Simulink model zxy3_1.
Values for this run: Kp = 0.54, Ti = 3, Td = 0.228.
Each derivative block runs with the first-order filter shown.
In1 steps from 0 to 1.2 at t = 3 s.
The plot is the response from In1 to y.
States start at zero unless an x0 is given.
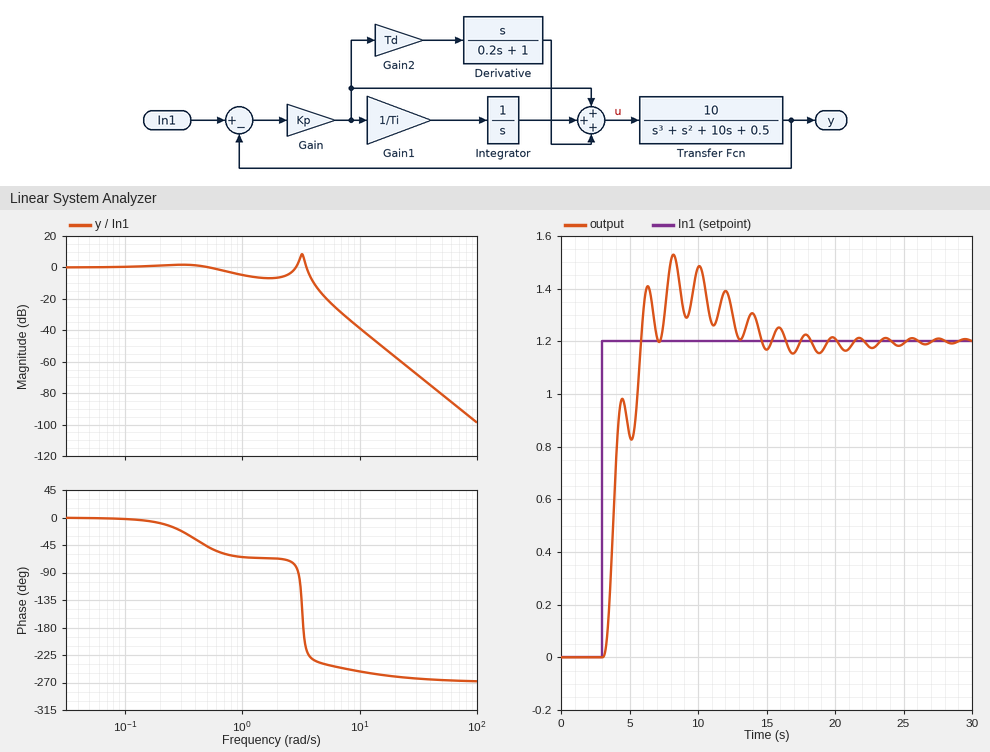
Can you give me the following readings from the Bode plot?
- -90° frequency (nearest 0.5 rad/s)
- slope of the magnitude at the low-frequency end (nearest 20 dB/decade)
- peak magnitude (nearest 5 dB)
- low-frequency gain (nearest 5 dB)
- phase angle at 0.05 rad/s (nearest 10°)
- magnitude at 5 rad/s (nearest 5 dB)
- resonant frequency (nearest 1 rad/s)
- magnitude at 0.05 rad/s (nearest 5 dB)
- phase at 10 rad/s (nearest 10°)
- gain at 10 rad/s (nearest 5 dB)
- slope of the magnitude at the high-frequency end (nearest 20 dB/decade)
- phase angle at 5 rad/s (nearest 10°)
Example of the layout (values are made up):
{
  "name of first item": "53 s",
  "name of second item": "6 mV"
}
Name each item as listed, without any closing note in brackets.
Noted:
{
  "-90° frequency": "3.0 rad/s",
  "slope of the magnitude at the low-frequency end": "0 dB/decade",
  "peak magnitude": "10 dB",
  "low-frequency gain": "0 dB",
  "phase angle at 0.05 rad/s": "0°",
  "magnitude at 5 rad/s": "-20 dB",
  "resonant frequency": "3 rad/s",
  "magnitude at 0.05 rad/s": "0 dB",
  "phase at 10 rad/s": "-250°",
  "gain at 10 rad/s": "-40 dB",
  "slope of the magnitude at the high-frequency end": "-60 dB/decade",
  "phase angle at 5 rad/s": "-240°"
}
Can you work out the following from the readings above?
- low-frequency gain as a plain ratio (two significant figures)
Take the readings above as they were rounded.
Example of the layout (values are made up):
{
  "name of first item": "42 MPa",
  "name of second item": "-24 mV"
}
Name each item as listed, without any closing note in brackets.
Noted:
{
  "low-frequency gain as a plain ratio": "1.0"
}
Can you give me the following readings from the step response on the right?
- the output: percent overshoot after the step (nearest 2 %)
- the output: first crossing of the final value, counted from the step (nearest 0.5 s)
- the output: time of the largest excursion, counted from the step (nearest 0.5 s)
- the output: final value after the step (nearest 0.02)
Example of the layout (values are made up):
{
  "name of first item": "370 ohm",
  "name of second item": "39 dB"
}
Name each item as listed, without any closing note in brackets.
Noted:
{
  "the output: percent overshoot after the step": "28 %",
  "the output: first crossing of the final value, counted from the step": "3.0 s",
  "the output: time of the largest excursion, counted from the step": "5.0 s",
  "the output: final value after the step": "1.20"
}
